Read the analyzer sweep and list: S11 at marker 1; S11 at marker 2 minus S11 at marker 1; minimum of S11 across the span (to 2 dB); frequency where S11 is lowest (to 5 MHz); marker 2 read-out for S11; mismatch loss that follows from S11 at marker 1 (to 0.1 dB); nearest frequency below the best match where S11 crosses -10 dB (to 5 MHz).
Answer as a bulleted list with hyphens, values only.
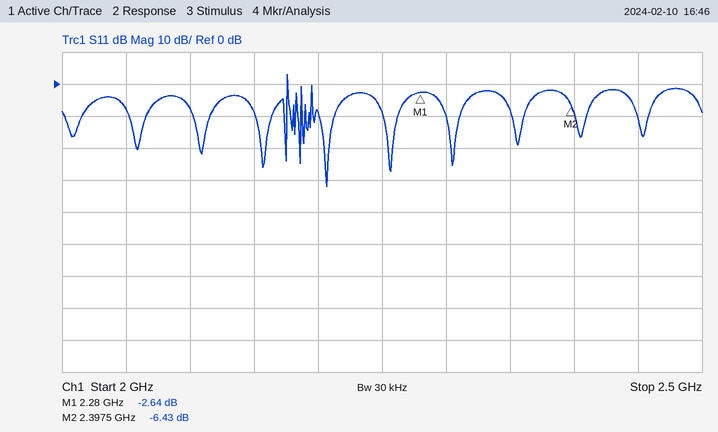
- -2.64 dB
- -3.79 dB
- -32 dB
- 2.205 GHz
- -6.43 dB
- 3.4 dB
- 2.200 GHz
